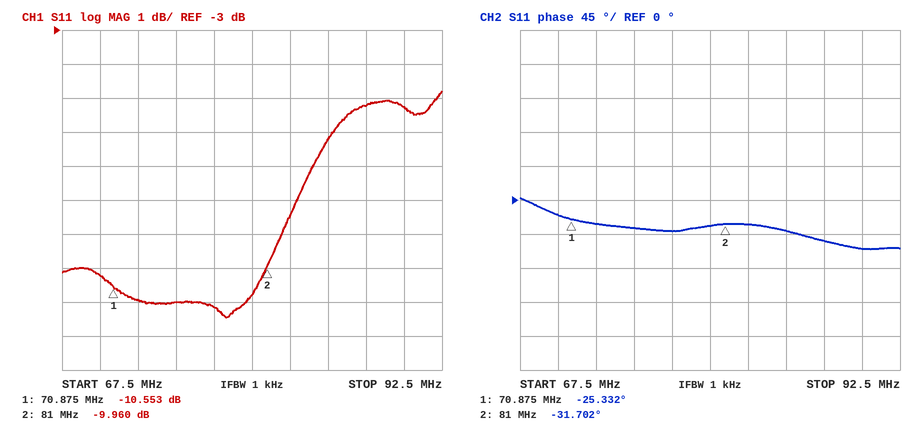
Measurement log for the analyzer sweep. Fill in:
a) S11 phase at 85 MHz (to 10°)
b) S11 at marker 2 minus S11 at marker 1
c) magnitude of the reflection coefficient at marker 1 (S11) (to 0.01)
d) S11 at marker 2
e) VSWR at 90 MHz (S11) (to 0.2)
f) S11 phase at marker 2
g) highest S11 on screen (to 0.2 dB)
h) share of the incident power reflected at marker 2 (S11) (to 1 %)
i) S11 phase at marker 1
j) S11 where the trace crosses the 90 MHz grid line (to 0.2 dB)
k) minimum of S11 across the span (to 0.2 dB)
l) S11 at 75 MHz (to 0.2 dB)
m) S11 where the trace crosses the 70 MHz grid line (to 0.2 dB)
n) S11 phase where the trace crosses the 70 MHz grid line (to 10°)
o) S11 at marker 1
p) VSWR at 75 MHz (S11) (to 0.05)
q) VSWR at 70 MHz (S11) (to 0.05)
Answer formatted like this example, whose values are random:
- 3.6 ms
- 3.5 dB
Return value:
- -40°
- 0.593 dB
- 0.30
- -9.960 dB
- 3.4
- -31.702°
- -4.8 dB
- 10 %
- -25.332°
- -5.2 dB
- -11.4 dB
- -11.0 dB
- -10.2 dB
- -20°
- -10.553 dB
- 1.80
- 1.90
